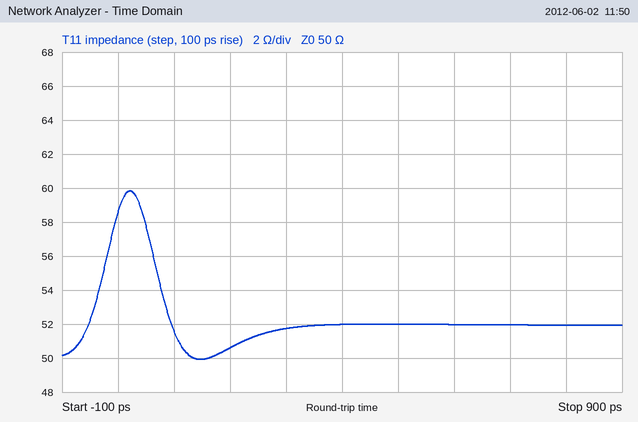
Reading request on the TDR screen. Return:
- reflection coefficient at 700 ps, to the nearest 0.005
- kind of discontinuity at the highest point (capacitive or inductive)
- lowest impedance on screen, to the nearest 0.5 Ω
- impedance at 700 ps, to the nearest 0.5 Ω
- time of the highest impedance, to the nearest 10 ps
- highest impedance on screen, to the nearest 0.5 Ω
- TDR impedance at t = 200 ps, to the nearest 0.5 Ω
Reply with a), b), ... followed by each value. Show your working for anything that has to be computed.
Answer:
a) (52 − 50)/(52 + 50) ≈ +0.020
b) inductive
c) 50.0 Ω
d) 52.0 Ω
e) 20 ps
f) 60.0 Ω
g) 50.5 Ω
